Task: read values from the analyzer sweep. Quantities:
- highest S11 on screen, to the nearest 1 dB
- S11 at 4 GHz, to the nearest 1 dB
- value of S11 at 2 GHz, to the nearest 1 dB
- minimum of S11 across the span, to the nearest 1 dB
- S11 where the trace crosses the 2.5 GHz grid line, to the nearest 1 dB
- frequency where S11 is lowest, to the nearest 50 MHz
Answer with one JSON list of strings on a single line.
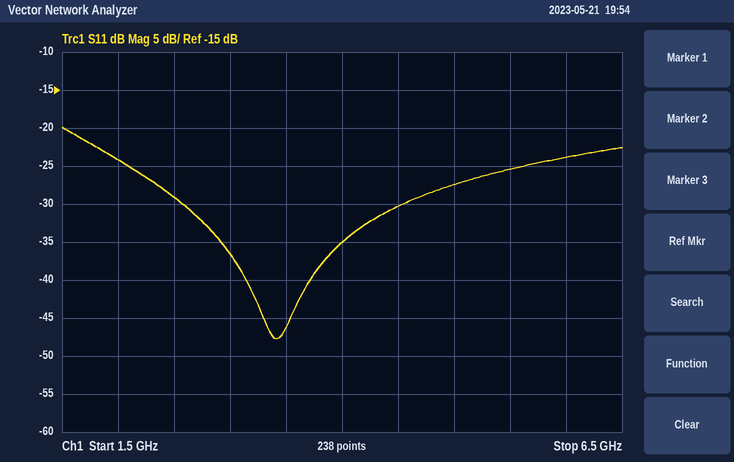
["-20 dB", "-35 dB", "-24 dB", "-48 dB", "-29 dB", "3.40 GHz"]
